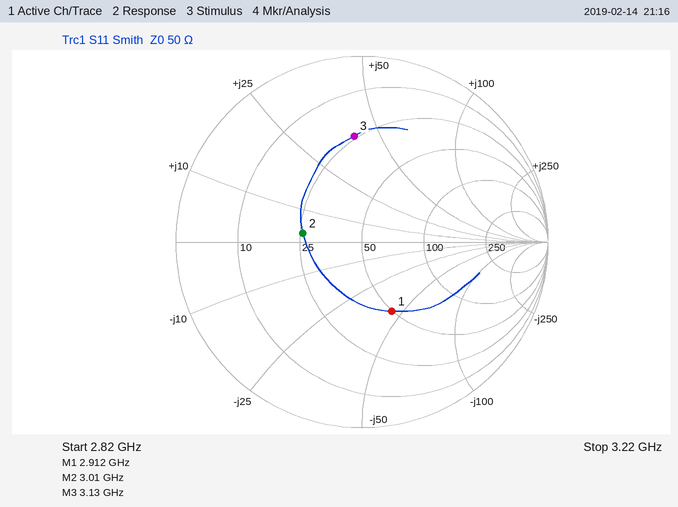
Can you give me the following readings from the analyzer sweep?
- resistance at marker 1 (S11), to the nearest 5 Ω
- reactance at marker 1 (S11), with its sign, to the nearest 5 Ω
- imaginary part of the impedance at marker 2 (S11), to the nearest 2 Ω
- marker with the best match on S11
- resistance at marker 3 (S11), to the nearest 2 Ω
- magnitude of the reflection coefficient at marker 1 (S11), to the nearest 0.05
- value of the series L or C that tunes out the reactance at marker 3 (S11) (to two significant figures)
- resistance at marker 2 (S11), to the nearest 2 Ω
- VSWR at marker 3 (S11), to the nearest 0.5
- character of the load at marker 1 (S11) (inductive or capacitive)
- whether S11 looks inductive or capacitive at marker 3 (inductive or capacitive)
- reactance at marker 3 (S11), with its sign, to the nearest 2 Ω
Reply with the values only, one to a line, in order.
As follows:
50 Ω
-45 Ω
+2 Ω
marker 2
24 Ω
0.40
1.3 pF
26 Ω
3.5
capacitive
inductive
+40 Ω
